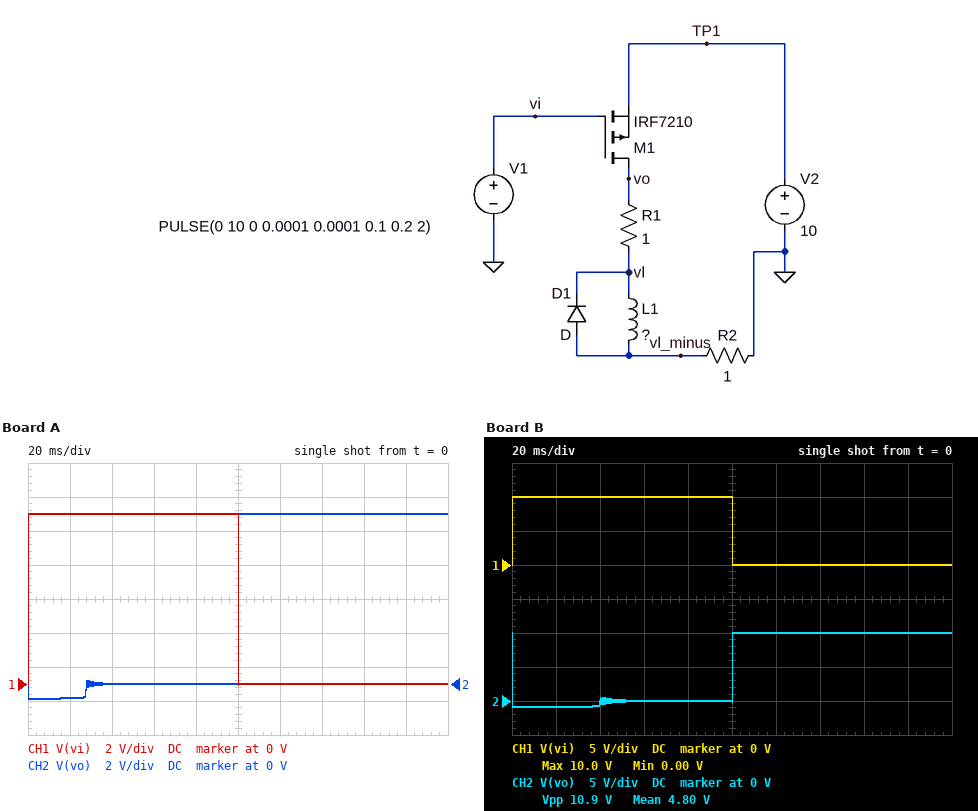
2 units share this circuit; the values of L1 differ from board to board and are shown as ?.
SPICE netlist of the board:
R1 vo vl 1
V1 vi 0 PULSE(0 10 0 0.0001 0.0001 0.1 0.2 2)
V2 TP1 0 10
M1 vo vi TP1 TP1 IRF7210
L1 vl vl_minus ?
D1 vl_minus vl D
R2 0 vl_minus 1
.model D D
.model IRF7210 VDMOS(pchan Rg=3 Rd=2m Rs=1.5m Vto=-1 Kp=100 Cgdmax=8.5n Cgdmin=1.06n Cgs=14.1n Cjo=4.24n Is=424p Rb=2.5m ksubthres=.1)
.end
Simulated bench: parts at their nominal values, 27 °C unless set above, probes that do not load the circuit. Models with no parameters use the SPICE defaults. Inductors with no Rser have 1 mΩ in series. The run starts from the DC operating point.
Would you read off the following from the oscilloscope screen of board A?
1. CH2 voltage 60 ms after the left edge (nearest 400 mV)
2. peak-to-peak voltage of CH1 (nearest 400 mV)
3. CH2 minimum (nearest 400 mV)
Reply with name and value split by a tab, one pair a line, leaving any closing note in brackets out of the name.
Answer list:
CH2 voltage 60 ms after the left edge	0 V
peak-to-peak voltage of CH1	10.0 V
CH2 minimum	-800 mV
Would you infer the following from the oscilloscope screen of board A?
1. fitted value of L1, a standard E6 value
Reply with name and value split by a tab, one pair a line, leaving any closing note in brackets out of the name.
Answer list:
fitted value of L1, a standard E6 value	4.7 mH
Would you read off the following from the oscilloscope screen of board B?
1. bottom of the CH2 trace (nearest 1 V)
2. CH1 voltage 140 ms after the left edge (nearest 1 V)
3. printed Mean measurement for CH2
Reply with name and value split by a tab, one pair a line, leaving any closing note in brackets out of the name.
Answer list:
bottom of the CH2 trace	-1 V
CH1 voltage 140 ms after the left edge	0 V
printed Mean measurement for CH2	4.80 V
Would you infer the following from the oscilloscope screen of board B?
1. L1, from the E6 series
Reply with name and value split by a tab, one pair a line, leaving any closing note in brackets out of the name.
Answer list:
L1, from the E6 series	6.8 mH
